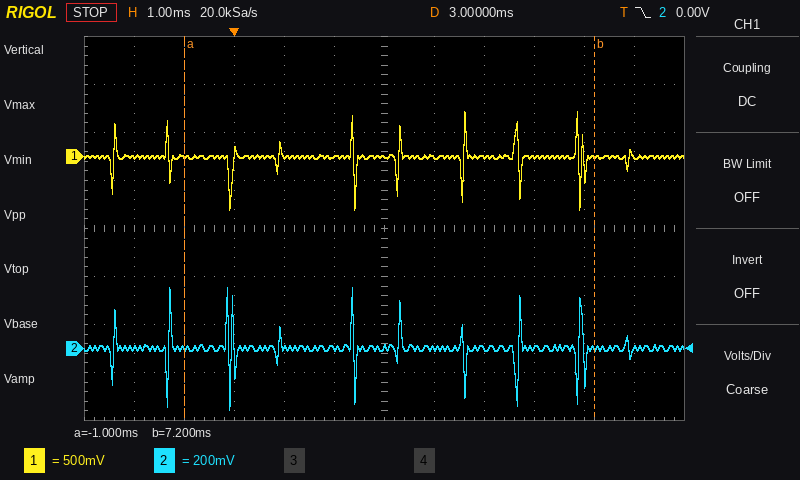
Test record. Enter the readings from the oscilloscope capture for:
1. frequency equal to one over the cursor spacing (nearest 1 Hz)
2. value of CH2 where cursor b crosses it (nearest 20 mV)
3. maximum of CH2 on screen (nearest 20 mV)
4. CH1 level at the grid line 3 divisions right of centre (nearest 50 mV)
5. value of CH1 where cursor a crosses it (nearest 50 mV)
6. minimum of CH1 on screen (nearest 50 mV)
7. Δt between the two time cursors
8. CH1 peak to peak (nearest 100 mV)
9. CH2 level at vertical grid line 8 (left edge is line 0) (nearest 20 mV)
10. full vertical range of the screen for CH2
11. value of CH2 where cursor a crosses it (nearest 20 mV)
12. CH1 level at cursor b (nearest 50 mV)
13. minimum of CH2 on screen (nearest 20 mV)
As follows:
122 Hz
0 mV
260 mV
0 mV
0 mV
-550 mV
8.2 ms
1.00 V
0 mV
1.6 V
0 mV
0 mV
-260 mV
